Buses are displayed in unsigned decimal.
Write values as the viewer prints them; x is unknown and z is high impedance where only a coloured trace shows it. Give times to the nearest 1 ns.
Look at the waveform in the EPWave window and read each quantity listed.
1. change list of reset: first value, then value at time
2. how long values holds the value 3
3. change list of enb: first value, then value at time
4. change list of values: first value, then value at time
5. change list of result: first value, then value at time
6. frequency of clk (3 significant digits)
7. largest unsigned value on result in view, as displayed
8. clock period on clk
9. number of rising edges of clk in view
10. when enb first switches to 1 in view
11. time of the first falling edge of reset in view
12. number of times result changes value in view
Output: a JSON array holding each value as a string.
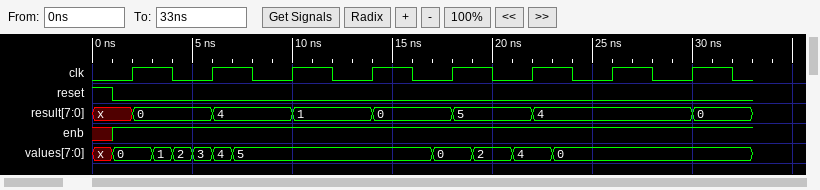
["1, 0 at 1 ns", "1 ns", "x, 1 at 1 ns", "x, 0 at 1 ns, 1 at 3 ns, 2 at 4 ns, 3 at 5 ns, 4 at 6 ns, 5 at 7 ns, 0 at 17 ns, 2 at 19 ns, 4 at 21 ns, 0 at 23 ns", "x, 0 at 2 ns, 4 at 6 ns, 1 at 10 ns, 0 at 14 ns, 5 at 18 ns, 4 at 22 ns, 0 at 30 ns", "250 MHz", "5", "4 ns", "8", "1 ns", "1 ns", "7"]
